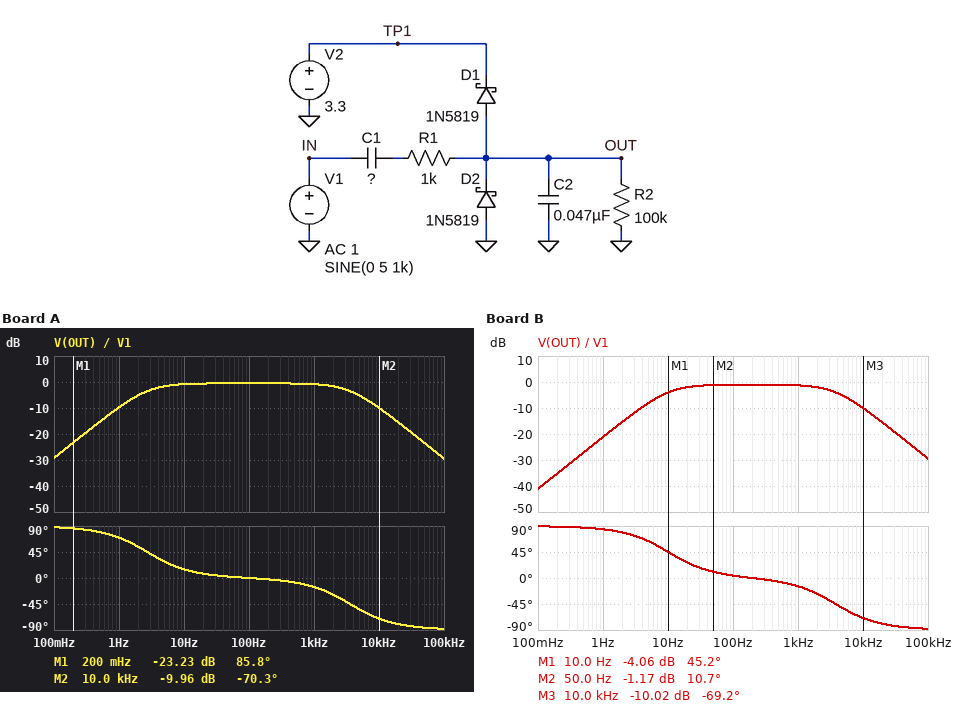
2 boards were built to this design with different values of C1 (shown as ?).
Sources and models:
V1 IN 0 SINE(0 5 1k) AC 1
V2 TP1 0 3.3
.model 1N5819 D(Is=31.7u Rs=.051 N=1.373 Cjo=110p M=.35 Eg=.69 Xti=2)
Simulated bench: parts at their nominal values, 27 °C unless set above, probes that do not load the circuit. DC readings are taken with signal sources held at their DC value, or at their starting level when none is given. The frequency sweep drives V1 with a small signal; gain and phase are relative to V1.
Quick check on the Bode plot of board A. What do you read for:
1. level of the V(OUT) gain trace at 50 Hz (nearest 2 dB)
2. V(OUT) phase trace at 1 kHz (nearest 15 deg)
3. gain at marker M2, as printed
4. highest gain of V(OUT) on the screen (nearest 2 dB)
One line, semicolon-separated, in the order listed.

0 dB; -15 deg; -9.96 dB; 0 dB
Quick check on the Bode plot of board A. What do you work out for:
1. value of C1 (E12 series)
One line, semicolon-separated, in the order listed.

2.2 µF
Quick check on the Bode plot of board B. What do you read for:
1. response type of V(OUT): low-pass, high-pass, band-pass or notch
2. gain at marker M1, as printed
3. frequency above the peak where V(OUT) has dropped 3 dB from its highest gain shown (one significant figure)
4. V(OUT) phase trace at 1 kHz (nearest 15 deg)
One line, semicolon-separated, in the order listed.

band-pass; -4.06 dB; 4 kHz; -15 deg
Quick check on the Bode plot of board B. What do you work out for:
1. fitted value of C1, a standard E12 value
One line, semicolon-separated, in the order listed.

560 nF
